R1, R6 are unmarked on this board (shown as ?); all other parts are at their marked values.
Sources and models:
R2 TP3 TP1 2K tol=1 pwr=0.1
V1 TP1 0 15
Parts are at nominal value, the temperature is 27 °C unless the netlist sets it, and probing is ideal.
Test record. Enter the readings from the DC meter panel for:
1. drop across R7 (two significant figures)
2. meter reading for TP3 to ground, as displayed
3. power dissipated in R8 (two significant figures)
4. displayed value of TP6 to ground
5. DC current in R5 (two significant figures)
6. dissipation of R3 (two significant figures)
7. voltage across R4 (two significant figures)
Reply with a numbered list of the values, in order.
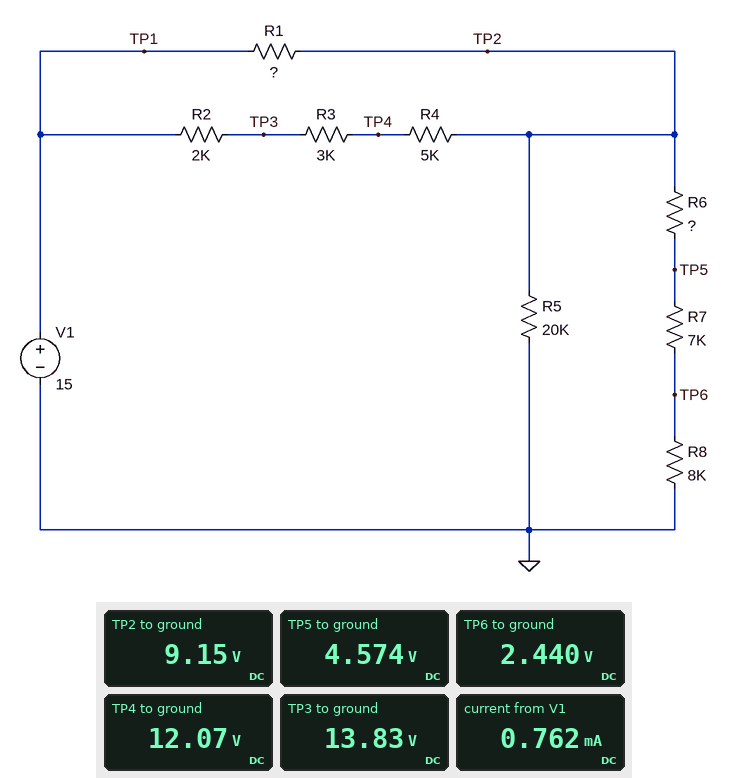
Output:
1. 2.1 V
2. 13.83 V
3. 740 µW
4. 2.440 V
5. 460 µA
6. 1.0 mW
7. 2.9 V
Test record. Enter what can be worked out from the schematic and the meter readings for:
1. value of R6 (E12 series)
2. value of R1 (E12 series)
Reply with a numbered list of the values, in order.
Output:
1. 15 kΩ
2. 33 kΩ
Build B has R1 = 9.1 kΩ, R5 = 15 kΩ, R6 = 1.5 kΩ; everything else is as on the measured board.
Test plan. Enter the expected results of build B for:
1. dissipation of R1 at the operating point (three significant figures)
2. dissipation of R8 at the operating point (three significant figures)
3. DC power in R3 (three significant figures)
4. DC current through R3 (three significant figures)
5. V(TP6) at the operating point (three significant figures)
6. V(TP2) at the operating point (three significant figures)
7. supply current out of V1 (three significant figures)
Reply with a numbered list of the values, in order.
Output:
1. 3.52 mW
2. 2.56 mW
3. 962 µW
4. 566 µA
5. 4.53 V
6. 9.34 V
7. 1.19 mA
